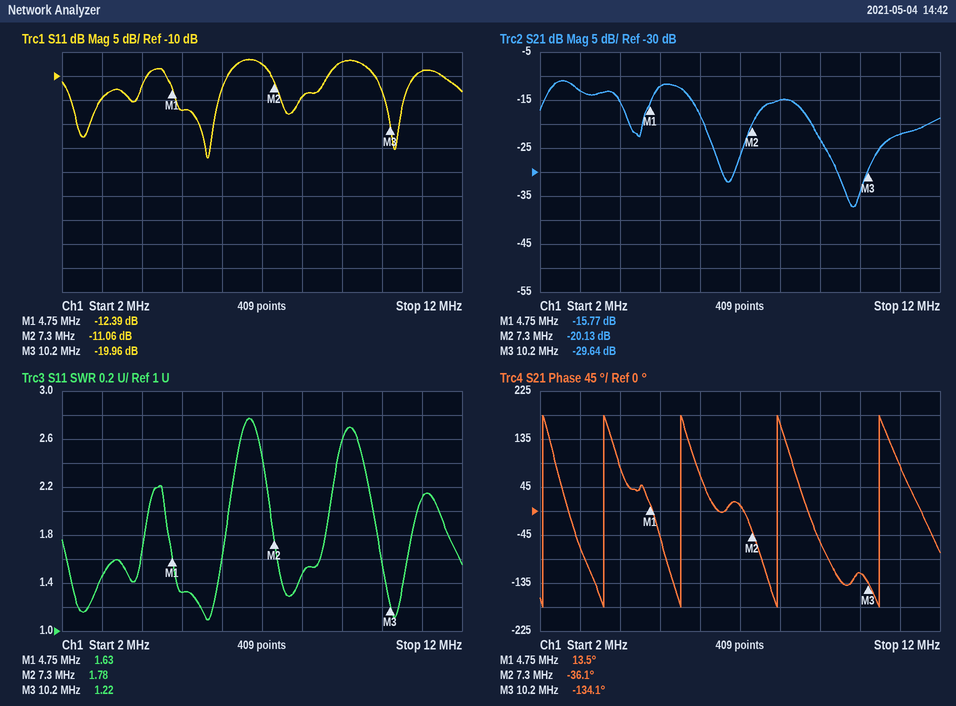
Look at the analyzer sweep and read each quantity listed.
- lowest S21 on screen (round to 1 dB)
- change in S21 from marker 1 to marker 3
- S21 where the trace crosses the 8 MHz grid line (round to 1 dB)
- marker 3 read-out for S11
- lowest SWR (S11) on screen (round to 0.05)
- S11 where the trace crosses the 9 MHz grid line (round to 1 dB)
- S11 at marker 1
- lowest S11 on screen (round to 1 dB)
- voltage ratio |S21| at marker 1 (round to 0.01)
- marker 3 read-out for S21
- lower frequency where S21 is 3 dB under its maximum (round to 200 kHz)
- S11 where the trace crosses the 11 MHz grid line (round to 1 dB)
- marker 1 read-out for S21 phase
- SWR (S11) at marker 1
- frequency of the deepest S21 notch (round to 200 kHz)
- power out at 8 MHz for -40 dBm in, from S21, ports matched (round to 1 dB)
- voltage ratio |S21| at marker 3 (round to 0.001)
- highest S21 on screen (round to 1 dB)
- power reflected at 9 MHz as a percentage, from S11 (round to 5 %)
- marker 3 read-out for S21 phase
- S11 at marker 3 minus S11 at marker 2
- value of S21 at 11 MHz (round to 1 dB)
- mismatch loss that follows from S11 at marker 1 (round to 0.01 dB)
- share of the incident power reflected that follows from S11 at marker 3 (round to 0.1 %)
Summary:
-37 dB
-13.87 dB
-15 dB
-19.96 dB
1.10
-7 dB
-12.39 dB
-27 dB
0.16
-29.64 dB
2.2 MHz
-9 dB
13.5°
1.63
9.8 MHz
-55 dBm
0.033
-11 dB
20 %
-134.1°
-8.90 dB
-22 dB
0.26 dB
1.0 %
